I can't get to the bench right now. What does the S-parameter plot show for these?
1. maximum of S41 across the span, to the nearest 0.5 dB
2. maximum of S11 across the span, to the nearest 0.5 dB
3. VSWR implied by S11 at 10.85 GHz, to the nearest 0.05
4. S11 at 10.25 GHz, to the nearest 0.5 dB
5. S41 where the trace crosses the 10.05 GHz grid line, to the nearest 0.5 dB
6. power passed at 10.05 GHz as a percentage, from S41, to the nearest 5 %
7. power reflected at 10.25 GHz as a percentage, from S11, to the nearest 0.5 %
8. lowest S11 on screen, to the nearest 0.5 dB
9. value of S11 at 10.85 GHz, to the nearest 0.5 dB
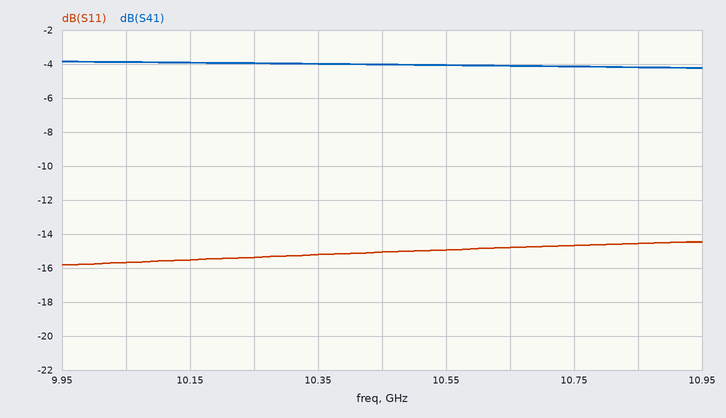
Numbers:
-4.0 dB
-14.5 dB
1.45
-15.5 dB
-4.0 dB
40 %
3.0 %
-16.0 dB
-14.5 dB
